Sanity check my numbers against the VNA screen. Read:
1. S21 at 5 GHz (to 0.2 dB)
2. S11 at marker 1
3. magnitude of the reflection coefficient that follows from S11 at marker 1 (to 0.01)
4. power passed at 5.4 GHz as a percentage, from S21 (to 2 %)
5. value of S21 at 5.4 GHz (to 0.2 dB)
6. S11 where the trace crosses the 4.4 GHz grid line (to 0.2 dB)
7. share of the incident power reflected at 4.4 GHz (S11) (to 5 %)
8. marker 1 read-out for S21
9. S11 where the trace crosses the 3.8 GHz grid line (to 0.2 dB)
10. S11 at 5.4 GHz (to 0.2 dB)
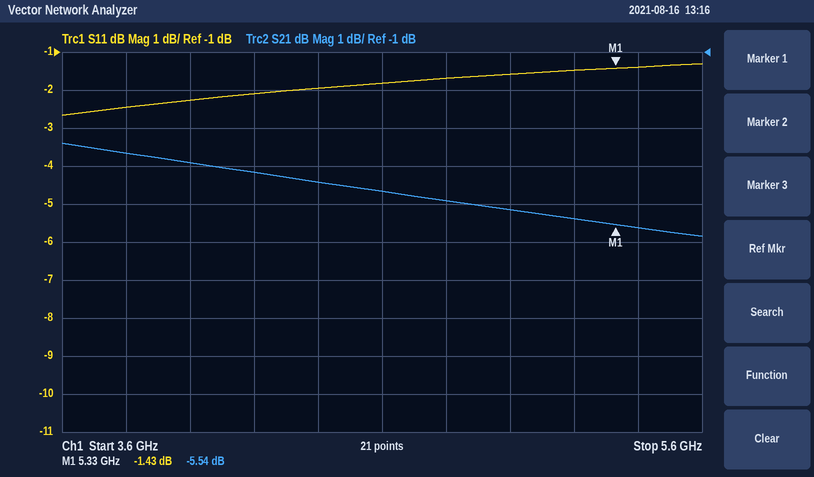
-5.2 dB
-1.43 dB
0.85
28 %
-5.6 dB
-2.0 dB
65 %
-5.54 dB
-2.4 dB
-1.4 dB
